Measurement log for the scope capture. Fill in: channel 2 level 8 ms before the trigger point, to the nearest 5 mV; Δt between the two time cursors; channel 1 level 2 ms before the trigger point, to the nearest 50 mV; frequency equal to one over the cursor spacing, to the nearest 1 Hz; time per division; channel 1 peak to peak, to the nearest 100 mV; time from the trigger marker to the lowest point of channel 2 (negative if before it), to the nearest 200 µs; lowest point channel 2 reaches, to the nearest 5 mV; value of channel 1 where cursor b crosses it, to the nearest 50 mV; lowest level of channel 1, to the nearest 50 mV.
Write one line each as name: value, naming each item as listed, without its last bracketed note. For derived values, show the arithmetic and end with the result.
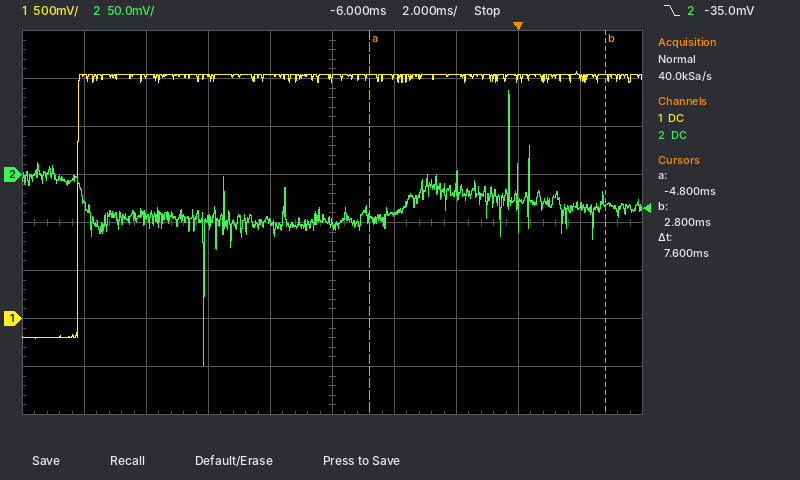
channel 2 level 8 ms before the trigger point, to the nearest 5 mV: -50 mV
Δt between the two time cursors: 7.6 ms
channel 1 level 2 ms before the trigger point, to the nearest 50 mV: 2.55 V
frequency equal to one over the cursor spacing, to the nearest 1 Hz: 1 / 7.6 ms ≈ 132 Hz
time per division: 2 ms
channel 1 peak to peak, to the nearest 100 mV: 2.80 V
time from the trigger marker to the lowest point of channel 2 (negative if before it), to the nearest 200 µs: -10.2 ms
lowest point channel 2 reaches, to the nearest 5 mV: -200 mV
value of channel 1 where cursor b crosses it, to the nearest 50 mV: 2.50 V
lowest level of channel 1, to the nearest 50 mV: -200 mV
